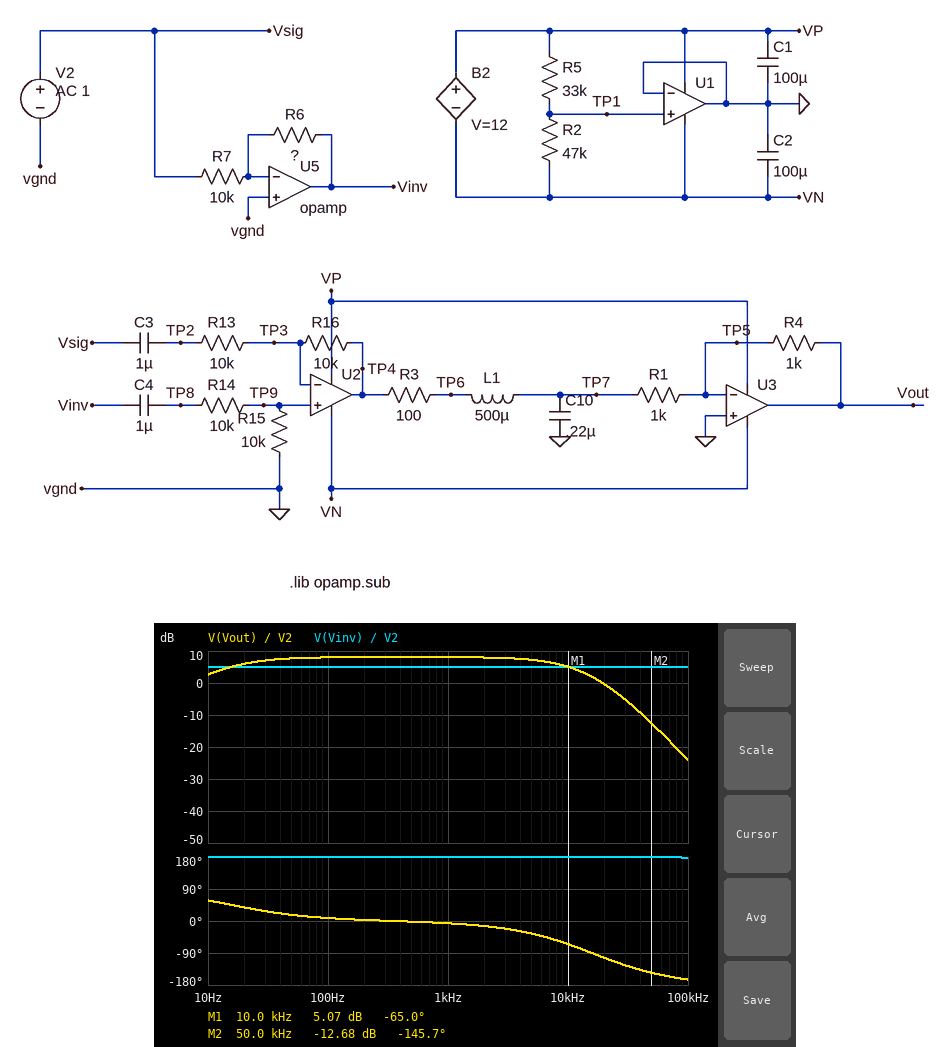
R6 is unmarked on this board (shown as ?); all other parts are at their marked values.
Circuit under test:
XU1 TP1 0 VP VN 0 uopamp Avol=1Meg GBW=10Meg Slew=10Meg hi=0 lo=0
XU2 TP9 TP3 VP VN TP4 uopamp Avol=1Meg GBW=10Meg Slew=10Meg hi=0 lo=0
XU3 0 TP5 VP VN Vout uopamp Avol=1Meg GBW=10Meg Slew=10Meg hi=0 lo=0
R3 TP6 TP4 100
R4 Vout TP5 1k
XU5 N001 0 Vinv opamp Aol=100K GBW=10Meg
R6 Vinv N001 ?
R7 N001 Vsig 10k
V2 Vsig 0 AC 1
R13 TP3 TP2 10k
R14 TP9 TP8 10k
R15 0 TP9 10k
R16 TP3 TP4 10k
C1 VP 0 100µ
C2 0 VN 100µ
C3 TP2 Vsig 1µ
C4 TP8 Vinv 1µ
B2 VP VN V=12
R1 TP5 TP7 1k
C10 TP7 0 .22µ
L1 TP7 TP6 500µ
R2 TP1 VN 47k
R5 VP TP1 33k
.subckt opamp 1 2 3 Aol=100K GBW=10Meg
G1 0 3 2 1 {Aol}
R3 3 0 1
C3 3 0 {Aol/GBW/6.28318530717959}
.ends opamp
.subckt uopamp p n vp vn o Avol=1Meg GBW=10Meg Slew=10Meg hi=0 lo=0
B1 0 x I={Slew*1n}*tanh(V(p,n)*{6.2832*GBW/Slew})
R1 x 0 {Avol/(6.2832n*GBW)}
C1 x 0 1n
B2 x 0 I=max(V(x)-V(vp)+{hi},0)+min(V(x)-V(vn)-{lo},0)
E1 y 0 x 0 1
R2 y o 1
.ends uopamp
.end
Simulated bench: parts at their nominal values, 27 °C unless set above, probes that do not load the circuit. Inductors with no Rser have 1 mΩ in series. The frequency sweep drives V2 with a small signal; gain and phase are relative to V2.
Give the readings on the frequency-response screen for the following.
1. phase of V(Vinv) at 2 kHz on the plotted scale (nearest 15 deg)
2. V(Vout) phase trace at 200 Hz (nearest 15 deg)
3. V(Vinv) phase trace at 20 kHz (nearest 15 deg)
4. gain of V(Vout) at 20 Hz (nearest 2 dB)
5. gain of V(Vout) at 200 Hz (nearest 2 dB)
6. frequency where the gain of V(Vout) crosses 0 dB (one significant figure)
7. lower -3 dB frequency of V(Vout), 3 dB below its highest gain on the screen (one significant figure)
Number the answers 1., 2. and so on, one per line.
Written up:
1. 180 deg
2. 0 deg
3. 180 deg
4. 6 dB
5. 8 dB
6. 20 kHz
7. 20 Hz
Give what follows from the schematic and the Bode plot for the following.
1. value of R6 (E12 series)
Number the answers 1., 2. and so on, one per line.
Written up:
1. 18 kΩ
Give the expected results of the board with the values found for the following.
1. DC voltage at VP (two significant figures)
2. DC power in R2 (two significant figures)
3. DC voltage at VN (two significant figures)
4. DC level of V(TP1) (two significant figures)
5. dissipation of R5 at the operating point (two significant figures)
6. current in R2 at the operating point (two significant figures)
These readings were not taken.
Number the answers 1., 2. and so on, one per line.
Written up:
1. 8.5 V
2. 1.1 mW
3. -3.5 V
4. 3.5 V
5. 740 µW
6. 150 µA
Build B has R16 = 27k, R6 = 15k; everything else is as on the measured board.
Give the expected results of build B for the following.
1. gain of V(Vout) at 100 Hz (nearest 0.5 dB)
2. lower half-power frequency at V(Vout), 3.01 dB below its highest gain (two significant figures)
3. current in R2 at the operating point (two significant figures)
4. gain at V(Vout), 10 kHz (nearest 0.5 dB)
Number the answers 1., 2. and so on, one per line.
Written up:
1. 14.0 dB
2. 17 Hz
3. 150 µA
4. 11.0 dB
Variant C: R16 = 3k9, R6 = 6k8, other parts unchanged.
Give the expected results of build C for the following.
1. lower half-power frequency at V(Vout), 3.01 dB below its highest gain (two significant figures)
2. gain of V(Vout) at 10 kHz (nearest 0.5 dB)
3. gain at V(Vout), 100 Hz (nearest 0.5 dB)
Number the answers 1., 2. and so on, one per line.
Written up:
1. 14 Hz
2. -5.0 dB
3. -2.0 dB
